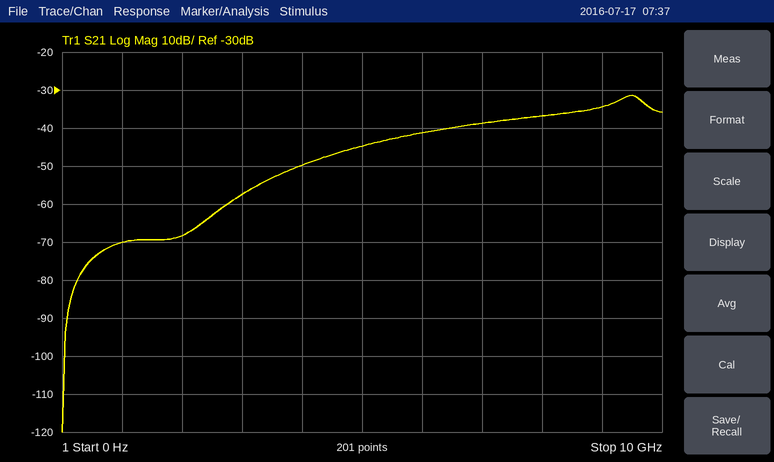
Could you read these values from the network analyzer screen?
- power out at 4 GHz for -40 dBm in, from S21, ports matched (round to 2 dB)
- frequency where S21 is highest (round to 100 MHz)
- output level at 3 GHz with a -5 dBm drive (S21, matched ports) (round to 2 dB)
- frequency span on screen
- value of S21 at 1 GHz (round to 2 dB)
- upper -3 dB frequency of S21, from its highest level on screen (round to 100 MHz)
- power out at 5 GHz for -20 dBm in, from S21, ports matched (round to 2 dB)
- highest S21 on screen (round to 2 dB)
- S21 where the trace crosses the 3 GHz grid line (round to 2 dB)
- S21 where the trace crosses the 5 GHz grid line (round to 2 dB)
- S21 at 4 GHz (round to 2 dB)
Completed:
-90 dBm
9.5 GHz
-62 dBm
10 GHz
-70 dB
9.8 GHz
-64 dBm
-32 dB
-58 dB
-44 dB
-50 dB
